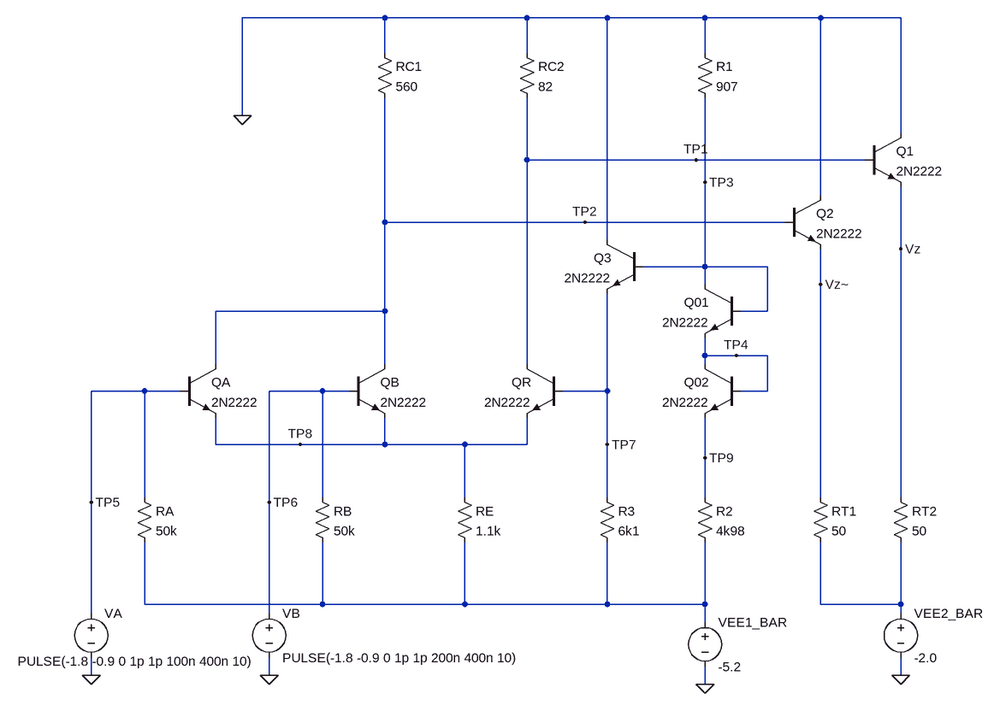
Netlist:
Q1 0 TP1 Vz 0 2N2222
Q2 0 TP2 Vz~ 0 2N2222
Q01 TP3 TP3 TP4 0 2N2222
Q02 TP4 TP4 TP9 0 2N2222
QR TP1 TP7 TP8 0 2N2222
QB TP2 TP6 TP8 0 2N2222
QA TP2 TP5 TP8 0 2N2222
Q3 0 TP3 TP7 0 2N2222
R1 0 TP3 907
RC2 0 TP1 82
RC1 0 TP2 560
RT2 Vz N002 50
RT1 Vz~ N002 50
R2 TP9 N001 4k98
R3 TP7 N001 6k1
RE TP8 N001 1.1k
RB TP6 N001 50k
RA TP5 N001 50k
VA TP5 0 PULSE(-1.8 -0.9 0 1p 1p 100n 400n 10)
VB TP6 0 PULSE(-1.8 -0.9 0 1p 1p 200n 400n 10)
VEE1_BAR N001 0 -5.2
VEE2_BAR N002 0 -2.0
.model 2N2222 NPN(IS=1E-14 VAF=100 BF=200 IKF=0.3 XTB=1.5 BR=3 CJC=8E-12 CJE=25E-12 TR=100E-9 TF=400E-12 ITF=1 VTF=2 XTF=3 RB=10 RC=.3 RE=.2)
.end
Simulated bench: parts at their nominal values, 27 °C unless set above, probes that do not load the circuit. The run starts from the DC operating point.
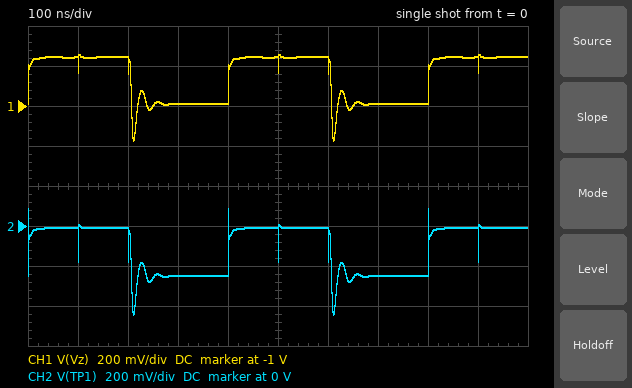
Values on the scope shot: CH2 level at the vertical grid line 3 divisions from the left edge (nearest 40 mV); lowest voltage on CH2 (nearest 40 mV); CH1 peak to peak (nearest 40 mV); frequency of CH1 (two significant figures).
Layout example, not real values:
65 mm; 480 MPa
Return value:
-240 mV; -440 mV; 440 mV; 2.5 MHz
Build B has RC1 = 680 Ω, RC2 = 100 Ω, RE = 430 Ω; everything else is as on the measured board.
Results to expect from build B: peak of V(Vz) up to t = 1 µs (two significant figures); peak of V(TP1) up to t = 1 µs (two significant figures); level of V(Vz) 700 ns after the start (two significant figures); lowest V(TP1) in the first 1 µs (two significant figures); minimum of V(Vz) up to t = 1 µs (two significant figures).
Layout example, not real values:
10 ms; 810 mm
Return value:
-760 mV; -9.6 mV; -1.5 V; -1.6 V; -2.1 V
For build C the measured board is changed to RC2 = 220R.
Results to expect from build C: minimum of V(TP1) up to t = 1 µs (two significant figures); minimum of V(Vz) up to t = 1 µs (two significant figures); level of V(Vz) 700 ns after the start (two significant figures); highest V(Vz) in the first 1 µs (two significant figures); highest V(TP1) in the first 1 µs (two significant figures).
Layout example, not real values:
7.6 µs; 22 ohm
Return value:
-890 mV; -1.6 V; -1.4 V; -760 mV; -16 mV
